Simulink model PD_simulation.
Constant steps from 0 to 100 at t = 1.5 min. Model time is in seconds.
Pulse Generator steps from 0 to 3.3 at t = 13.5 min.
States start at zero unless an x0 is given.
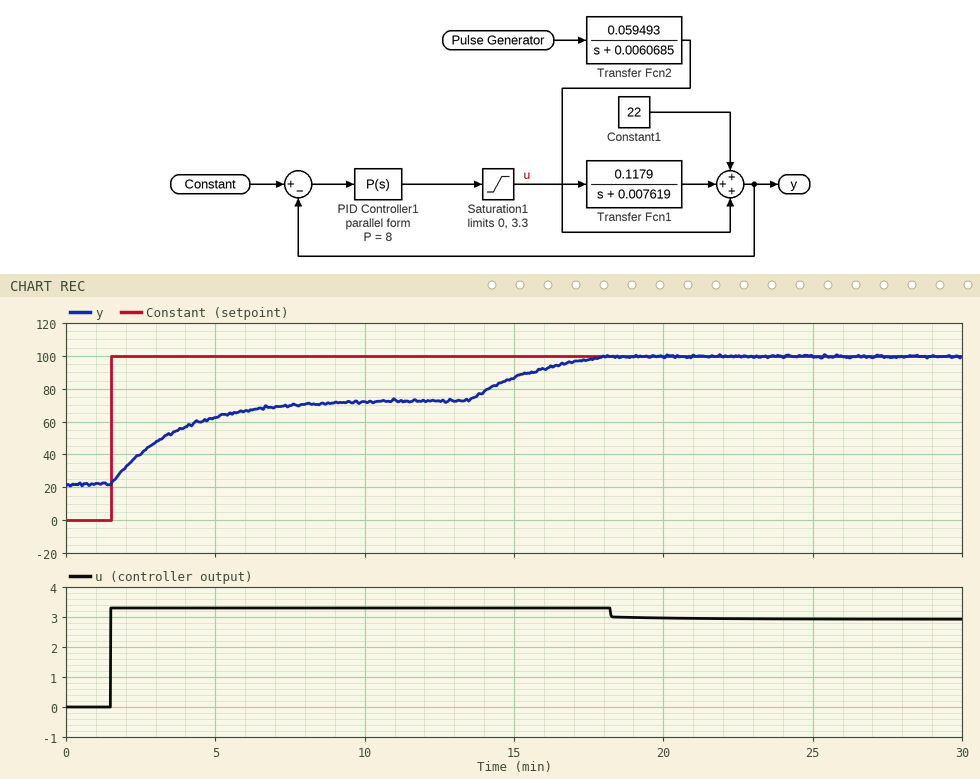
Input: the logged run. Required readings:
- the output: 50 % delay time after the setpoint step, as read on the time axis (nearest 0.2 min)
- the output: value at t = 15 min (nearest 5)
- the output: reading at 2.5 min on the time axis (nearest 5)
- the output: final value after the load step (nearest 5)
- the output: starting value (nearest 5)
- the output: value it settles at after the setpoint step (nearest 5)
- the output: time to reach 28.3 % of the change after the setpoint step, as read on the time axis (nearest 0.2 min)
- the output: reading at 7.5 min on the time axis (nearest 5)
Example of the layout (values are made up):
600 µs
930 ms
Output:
3.0 min
85
40
100
20
75
2.2 min
70
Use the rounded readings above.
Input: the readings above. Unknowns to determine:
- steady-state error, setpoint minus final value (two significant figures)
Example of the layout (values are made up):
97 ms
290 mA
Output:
25
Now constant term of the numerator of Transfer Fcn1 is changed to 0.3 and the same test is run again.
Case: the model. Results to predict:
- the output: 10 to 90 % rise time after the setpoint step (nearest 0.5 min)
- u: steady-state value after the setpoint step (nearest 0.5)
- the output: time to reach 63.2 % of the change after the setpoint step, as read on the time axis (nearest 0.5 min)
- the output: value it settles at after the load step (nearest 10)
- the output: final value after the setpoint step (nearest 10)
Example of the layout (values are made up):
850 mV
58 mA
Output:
1.5 min
2.0
2.5 min
100
100
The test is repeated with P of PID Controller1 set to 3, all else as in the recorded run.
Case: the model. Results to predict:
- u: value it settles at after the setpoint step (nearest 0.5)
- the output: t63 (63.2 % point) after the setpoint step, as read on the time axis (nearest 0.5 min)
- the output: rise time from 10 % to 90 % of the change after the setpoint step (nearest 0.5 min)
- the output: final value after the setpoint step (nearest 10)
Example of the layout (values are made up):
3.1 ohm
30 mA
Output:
3.5
3.5 min
5.0 min
70
